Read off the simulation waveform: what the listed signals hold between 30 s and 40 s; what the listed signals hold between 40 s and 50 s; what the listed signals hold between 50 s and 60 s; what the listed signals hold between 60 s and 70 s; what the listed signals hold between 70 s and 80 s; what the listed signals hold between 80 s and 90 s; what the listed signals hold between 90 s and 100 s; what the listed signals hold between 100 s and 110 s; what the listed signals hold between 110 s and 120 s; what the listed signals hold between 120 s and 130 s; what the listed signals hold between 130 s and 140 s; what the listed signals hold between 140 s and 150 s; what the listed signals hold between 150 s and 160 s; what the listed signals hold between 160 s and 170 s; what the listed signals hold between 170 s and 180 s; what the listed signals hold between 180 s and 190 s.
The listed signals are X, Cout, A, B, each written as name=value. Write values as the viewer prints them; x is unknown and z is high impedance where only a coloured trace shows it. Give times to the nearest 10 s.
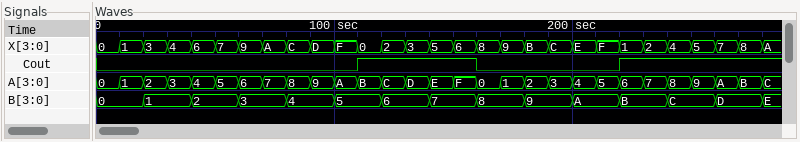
X=4, Cout=0, A=3, B=1
X=6, Cout=0, A=4, B=2
X=7, Cout=0, A=5, B=2
X=9, Cout=0, A=6, B=3
X=A, Cout=0, A=7, B=3
X=C, Cout=0, A=8, B=4
X=D, Cout=0, A=9, B=4
X=F, Cout=0, A=A, B=5
X=0, Cout=1, A=B, B=5
X=2, Cout=1, A=C, B=6
X=3, Cout=1, A=D, B=6
X=5, Cout=1, A=E, B=7
X=6, Cout=1, A=F, B=7
X=8, Cout=0, A=0, B=8
X=9, Cout=0, A=1, B=8
X=B, Cout=0, A=2, B=9
